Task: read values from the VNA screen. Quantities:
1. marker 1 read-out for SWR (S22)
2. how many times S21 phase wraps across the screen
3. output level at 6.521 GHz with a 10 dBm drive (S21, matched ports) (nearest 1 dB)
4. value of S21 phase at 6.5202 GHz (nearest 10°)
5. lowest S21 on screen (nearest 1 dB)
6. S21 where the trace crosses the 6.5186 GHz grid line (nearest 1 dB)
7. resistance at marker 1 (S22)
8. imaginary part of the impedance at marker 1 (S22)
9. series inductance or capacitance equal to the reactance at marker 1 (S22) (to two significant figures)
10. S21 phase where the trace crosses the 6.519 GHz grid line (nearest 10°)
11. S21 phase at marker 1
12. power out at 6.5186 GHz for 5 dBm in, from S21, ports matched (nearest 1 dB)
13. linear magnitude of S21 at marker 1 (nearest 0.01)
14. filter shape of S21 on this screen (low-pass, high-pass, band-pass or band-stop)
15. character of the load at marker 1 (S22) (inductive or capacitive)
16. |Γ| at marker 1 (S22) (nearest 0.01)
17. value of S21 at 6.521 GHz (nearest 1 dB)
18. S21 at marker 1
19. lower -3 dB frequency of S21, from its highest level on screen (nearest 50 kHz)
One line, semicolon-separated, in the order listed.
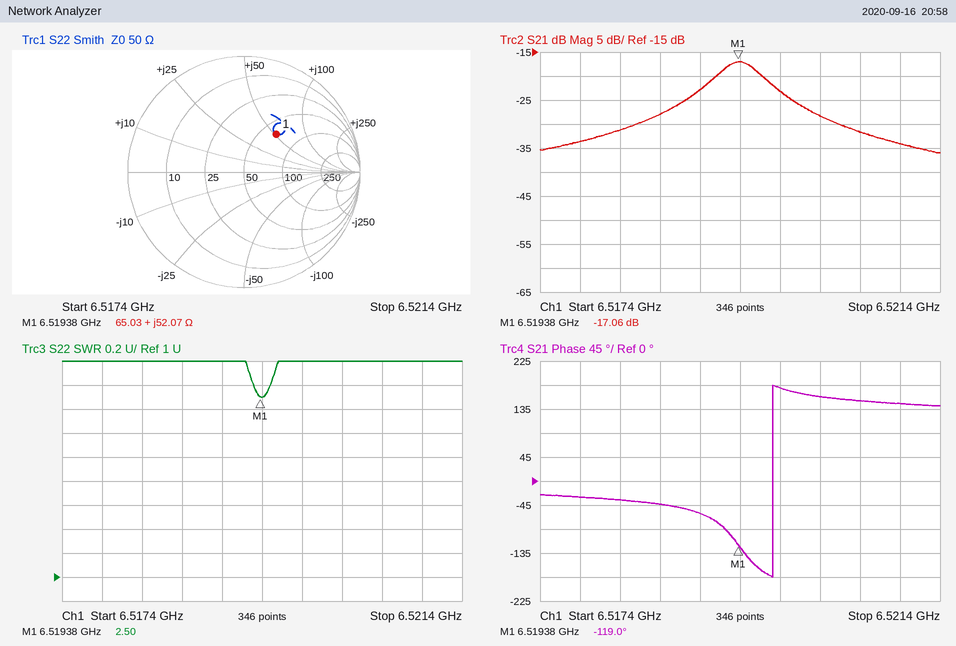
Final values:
2.50; 1; -24 dBm; 160°; -36 dB; -28 dB; 65.03 Ω; +52.07 Ω; 1.3 nH; -60°; -119.0°; -23 dBm; 0.14; band-pass; inductive; 0.43; -34 dB; -17.06 dB; 6.51915 GHz
